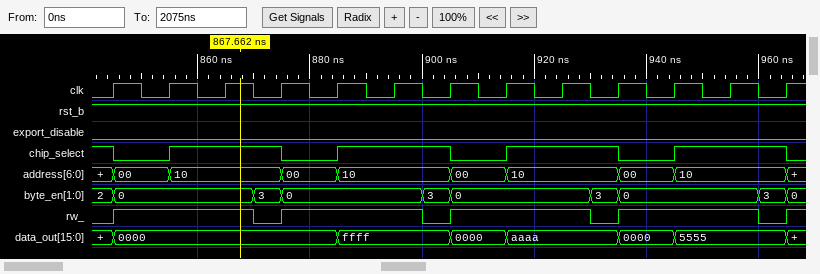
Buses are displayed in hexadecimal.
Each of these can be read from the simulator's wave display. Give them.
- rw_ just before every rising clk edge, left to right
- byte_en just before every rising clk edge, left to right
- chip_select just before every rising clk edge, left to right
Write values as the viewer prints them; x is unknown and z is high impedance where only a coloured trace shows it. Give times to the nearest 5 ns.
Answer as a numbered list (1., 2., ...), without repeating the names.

1. 0 1 1 0 1 1 0 1 1 0 1 1 0
2. 2, 0, 0, 3, 0, 0, 3, 0, 0, 3, 0, 0, 3
3. 1 0 1 1 0 1 1 0 1 1 0 1 1
